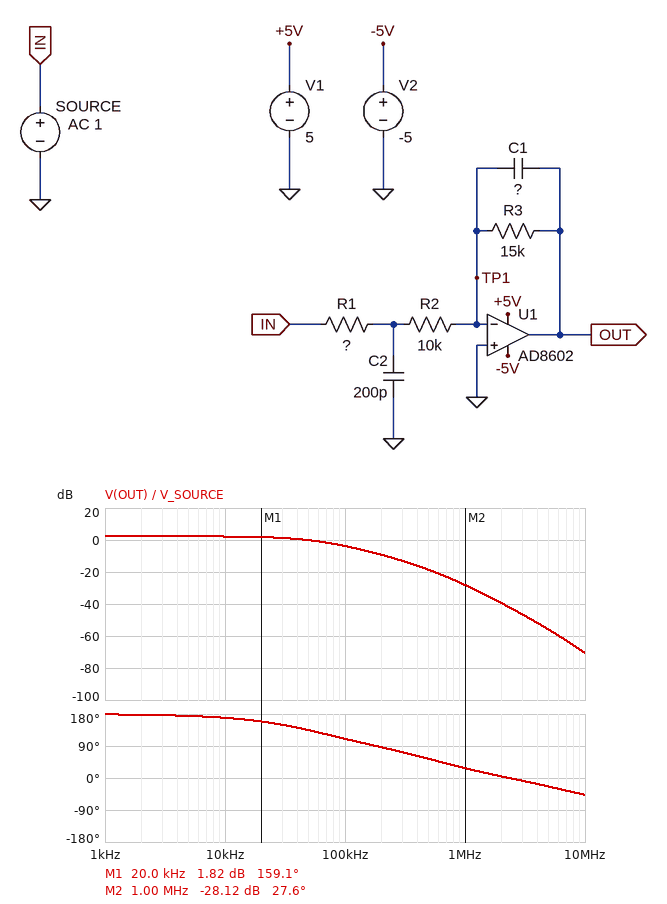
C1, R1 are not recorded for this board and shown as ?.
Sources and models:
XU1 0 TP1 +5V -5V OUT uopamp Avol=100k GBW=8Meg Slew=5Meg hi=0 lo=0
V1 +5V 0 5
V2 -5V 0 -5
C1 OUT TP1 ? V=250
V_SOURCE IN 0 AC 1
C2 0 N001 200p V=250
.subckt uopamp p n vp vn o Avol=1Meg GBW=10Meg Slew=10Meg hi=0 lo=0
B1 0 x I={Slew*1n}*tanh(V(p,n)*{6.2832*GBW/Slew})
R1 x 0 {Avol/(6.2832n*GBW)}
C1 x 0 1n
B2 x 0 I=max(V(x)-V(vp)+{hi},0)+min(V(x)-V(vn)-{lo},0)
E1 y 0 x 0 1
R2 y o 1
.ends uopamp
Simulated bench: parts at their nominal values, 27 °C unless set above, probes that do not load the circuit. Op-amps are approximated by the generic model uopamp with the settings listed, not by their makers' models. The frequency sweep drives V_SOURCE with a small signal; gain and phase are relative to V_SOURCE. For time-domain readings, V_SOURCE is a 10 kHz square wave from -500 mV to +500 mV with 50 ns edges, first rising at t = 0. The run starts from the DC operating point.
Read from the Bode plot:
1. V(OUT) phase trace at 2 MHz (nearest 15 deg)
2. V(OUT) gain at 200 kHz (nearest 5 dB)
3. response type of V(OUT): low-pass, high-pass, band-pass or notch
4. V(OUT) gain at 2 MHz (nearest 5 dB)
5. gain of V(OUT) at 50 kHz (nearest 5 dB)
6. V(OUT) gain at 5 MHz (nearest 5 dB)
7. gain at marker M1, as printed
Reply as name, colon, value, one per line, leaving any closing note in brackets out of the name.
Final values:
V(OUT) phase trace at 2 MHz: 0 deg
V(OUT) gain at 200 kHz: -10 dB
response type of V(OUT): low-pass, high-pass, band-pass or notch: low-pass
V(OUT) gain at 2 MHz: -40 dB
gain of V(OUT) at 50 kHz: 0 dB
V(OUT) gain at 5 MHz: -55 dB
gain at marker M1, as printed: 1.82 dB
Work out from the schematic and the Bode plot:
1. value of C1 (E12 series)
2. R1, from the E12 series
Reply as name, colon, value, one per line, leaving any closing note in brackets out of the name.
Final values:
value of C1: 180 pF
R1, from the E12 series: 1.5 kΩ
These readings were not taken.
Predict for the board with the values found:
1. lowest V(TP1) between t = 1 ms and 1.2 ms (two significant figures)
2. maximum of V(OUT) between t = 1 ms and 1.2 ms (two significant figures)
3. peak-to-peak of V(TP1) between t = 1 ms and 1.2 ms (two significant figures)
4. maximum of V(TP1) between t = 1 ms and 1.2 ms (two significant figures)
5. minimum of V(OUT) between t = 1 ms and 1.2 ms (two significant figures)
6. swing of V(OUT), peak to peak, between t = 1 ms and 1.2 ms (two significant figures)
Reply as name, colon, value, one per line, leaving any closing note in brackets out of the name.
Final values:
lowest V(TP1) between t = 1 ms and 1.2 ms: -7.5 mV
maximum of V(OUT) between t = 1 ms and 1.2 ms: 650 mV
peak-to-peak of V(TP1) between t = 1 ms and 1.2 ms: 15 mV
maximum of V(TP1) between t = 1 ms and 1.2 ms: 7.5 mV
minimum of V(OUT) between t = 1 ms and 1.2 ms: -650 mV
swing of V(OUT), peak to peak, between t = 1 ms and 1.2 ms: 1.3 V
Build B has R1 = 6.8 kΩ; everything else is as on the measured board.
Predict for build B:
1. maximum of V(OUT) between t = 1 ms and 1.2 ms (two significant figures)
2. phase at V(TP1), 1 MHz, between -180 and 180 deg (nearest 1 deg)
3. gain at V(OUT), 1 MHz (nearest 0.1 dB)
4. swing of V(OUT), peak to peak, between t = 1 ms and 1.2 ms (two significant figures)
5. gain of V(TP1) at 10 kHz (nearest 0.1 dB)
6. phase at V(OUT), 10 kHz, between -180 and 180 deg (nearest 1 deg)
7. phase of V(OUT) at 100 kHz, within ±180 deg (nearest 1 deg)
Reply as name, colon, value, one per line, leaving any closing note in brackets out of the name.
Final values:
maximum of V(OUT) between t = 1 ms and 1.2 ms: 450 mV
phase at V(TP1), 1 MHz, between -180 and 180 deg: -83 deg
gain at V(OUT), 1 MHz: -40.0 dB
swing of V(OUT), peak to peak, between t = 1 ms and 1.2 ms: 890 mV
gain of V(TP1) at 10 kHz: -59.2 dB
phase at V(OUT), 10 kHz, between -180 and 180 deg: 167 deg
phase of V(OUT) at 100 kHz, within ±180 deg: 93 deg
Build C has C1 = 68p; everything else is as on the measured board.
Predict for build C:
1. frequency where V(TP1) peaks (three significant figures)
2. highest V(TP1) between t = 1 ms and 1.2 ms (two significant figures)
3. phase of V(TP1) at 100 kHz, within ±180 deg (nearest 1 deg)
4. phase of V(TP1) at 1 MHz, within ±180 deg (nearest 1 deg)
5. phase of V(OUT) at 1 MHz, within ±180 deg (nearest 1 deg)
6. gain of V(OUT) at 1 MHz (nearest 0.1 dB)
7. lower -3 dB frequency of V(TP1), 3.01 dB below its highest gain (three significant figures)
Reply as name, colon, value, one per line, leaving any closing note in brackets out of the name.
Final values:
frequency where V(TP1) peaks: 303 kHz
highest V(TP1) between t = 1 ms and 1.2 ms: 16 mV
phase of V(TP1) at 100 kHz, within ±180 deg: 47 deg
phase of V(TP1) at 1 MHz, within ±180 deg: -57 deg
phase of V(OUT) at 1 MHz, within ±180 deg: 33 deg
gain of V(OUT) at 1 MHz: -19.9 dB
lower -3 dB frequency of V(TP1), 3.01 dB below its highest gain: 107 kHz
